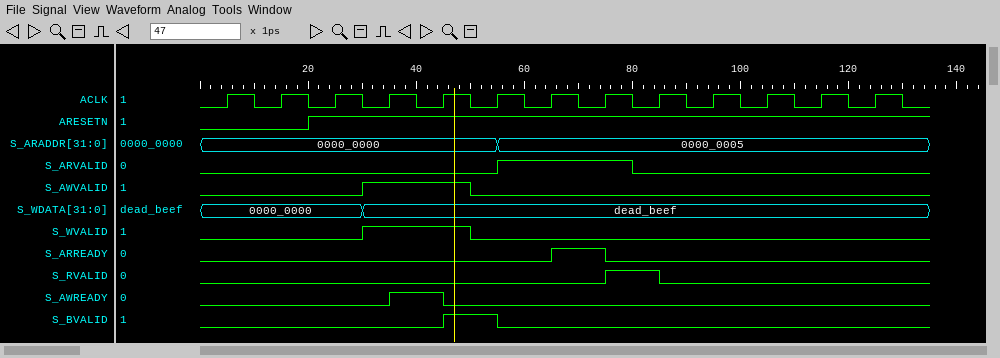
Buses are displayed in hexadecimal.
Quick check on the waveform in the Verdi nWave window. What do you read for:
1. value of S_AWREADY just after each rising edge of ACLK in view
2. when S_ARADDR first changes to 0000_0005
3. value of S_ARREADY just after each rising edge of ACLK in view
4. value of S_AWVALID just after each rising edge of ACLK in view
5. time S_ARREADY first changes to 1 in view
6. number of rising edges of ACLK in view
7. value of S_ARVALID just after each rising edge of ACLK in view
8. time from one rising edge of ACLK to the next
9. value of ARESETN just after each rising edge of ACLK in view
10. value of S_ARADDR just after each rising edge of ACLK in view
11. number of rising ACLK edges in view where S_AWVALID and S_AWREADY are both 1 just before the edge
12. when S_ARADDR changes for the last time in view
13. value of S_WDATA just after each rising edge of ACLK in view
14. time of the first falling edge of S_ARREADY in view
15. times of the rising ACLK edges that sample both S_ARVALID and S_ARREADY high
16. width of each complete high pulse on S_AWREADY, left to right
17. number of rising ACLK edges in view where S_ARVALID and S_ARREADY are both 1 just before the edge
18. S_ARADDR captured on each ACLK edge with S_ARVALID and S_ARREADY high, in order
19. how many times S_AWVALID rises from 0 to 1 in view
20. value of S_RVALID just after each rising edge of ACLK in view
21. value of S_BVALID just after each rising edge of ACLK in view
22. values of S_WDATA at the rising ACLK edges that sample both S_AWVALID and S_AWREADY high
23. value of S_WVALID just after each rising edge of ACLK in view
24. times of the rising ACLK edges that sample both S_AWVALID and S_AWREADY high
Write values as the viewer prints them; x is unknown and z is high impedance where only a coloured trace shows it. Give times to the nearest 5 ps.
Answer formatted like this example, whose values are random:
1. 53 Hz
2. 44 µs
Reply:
1. 0 0 0 1 0 0 0 0 0 0 0 0 0
2. 55 ps
3. 0 0 0 0 0 0 1 0 0 0 0 0 0
4. 0 0 0 1 1 0 0 0 0 0 0 0 0
5. 65 ps
6. 13
7. 0 0 0 0 0 1 1 1 0 0 0 0 0
8. 10 ps
9. 0 0 1 1 1 1 1 1 1 1 1 1 1
10. 0000_0000, 0000_0000, 0000_0000, 0000_0000, 0000_0000, 0000_0005, 0000_0005, 0000_0005, 0000_0005, 0000_0005, 0000_0005, 0000_0005, 0000_0005
11. 1
12. 55 ps
13. 0000_0000, 0000_0000, 0000_0000, dead_beef, dead_beef, dead_beef, dead_beef, dead_beef, dead_beef, dead_beef, dead_beef, dead_beef, dead_beef
14. 75 ps
15. 75 ps
16. 10 ps
17. 1
18. 0000_0005
19. 1
20. 0 0 0 0 0 0 0 1 0 0 0 0 0
21. 0 0 0 0 1 0 0 0 0 0 0 0 0
22. dead_beef
23. 0 0 0 1 1 0 0 0 0 0 0 0 0
24. 45 ps
